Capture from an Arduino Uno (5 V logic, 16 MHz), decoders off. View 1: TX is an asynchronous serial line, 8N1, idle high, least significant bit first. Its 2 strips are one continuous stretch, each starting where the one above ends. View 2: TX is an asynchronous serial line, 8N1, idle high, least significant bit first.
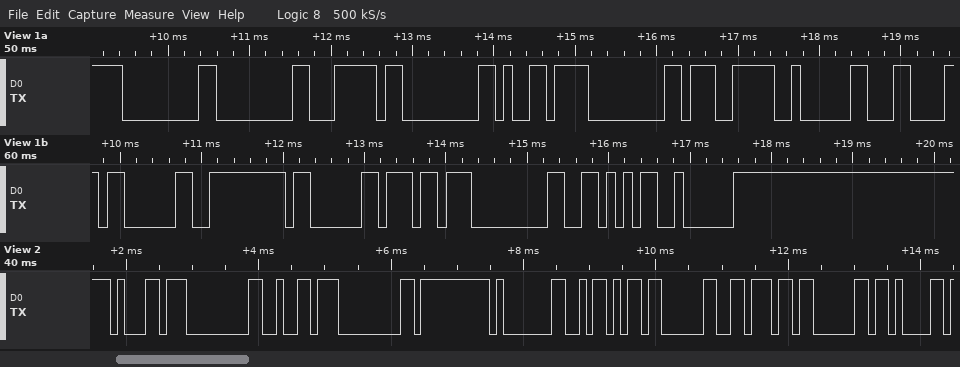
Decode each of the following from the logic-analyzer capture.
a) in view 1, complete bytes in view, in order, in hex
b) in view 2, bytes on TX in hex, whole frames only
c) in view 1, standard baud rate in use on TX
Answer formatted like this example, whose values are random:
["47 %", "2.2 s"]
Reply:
["00 00 7C 00 D9 00 E7 02 0C 03 FE 03 B7 00 56 02", "B1 00 B2 00 FF 01 5A 03 76 03 0B", "9600 baud"]
